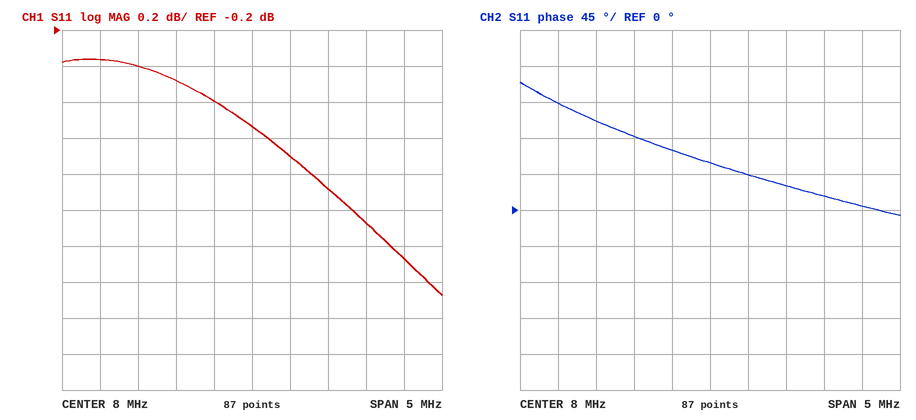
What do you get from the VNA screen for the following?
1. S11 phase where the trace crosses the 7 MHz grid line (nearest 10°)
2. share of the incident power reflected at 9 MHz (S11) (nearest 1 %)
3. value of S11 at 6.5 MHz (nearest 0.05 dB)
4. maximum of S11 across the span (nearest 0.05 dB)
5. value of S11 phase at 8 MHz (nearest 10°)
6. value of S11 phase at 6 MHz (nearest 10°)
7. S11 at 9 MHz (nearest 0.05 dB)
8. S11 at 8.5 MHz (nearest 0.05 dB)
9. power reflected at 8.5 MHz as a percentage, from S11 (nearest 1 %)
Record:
90°
78 %
-0.40 dB
-0.35 dB
60°
130°
-1.10 dB
-0.90 dB
81 %
